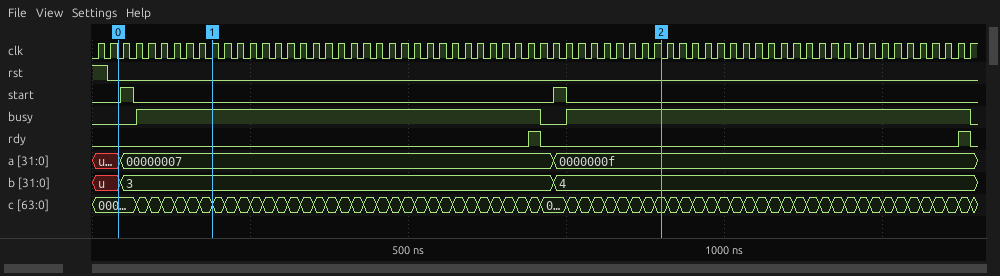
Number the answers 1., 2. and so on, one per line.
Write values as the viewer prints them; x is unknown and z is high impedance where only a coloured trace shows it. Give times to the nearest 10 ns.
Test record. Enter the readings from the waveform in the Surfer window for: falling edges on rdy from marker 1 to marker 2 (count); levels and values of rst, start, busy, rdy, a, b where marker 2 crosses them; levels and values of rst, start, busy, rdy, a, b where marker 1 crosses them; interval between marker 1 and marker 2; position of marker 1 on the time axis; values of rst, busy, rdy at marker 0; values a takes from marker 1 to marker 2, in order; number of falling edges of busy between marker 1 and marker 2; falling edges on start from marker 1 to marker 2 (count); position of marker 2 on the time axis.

1. 1
2. rst=0, start=0, busy=1, rdy=0, a=0000000f, b=4
3. rst=0, start=0, busy=1, rdy=0, a=00000007, b=3
4. 710 ns
5. 190 ns
6. rst=0, busy=0, rdy=0
7. 00000007, 0000000f
8. 1
9. 1
10. 900 ns
